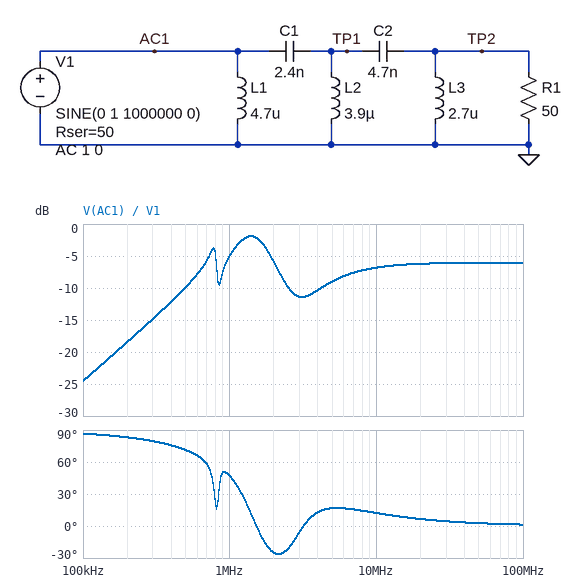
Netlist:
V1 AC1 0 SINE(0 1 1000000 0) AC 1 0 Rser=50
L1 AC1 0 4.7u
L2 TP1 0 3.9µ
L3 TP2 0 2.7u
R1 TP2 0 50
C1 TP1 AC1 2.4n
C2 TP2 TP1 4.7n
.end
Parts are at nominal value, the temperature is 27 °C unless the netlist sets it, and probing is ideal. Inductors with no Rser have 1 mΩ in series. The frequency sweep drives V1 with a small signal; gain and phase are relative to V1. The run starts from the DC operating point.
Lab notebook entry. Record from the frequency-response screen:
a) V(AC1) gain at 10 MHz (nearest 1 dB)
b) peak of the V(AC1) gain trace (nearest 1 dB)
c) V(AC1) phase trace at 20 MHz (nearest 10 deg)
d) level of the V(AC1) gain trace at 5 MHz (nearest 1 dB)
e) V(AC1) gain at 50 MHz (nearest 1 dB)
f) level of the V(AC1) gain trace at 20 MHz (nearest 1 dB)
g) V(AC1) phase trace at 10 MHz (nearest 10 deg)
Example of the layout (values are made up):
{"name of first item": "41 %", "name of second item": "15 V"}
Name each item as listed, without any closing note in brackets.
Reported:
{"V(AC1) gain at 10 MHz": "-7 dB", "peak of the V(AC1) gain trace": "-2 dB", "V(AC1) phase trace at 20 MHz": "10 deg", "level of the V(AC1) gain trace at 5 MHz": "-9 dB", "V(AC1) gain at 50 MHz": "-6 dB", "level of the V(AC1) gain trace at 20 MHz": "-6 dB", "V(AC1) phase trace at 10 MHz": "10 deg"}
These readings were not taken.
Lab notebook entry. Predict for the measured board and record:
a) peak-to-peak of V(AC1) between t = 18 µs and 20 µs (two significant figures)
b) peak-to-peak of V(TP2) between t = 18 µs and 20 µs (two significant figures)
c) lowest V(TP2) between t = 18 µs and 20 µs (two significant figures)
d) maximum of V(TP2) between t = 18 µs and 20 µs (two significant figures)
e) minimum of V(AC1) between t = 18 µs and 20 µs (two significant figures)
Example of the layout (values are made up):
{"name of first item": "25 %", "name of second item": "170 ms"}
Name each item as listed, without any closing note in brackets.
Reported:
{"peak-to-peak of V(AC1) between t = 18 µs and 20 µs": "1.1 V", "peak-to-peak of V(TP2) between t = 18 µs and 20 µs": "510 mV", "lowest V(TP2) between t = 18 µs and 20 µs": "-260 mV", "maximum of V(TP2) between t = 18 µs and 20 µs": "260 mV", "minimum of V(AC1) between t = 18 µs and 20 µs": "-570 mV"}
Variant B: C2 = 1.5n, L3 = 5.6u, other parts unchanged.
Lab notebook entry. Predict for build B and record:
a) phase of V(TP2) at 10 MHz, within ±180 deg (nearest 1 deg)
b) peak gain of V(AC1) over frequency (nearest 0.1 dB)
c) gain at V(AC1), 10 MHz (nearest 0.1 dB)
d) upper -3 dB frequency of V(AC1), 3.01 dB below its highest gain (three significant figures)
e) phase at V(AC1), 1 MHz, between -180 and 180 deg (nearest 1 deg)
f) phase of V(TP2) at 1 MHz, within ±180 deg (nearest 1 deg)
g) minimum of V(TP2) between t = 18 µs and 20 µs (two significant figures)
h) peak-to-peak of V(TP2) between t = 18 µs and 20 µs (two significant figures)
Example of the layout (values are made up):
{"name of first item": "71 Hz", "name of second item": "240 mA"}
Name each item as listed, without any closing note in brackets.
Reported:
{"phase of V(TP2) at 10 MHz, within ±180 deg": "25 deg", "peak gain of V(AC1) over frequency": "-1.1 dB", "gain at V(AC1), 10 MHz": "-6.2 dB", "upper -3 dB frequency of V(AC1), 3.01 dB below its highest gain": "1.08 MHz", "phase at V(AC1), 1 MHz, between -180 and 180 deg": "8 deg", "phase of V(TP2) at 1 MHz, within ±180 deg": "-48 deg", "minimum of V(TP2) between t = 18 µs and 20 µs": "-320 mV", "peak-to-peak of V(TP2) between t = 18 µs and 20 µs": "630 mV"}
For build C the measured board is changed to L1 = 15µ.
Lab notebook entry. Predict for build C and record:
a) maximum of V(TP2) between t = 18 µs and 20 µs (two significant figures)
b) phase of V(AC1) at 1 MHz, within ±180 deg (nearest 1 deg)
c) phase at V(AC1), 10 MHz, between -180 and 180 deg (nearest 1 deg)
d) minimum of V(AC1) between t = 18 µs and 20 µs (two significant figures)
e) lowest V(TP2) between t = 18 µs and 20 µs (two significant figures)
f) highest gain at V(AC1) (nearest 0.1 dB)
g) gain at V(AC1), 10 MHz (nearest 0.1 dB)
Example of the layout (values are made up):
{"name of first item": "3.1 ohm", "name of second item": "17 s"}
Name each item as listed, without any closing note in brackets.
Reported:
{"maximum of V(TP2) between t = 18 µs and 20 µs": "370 mV", "phase of V(AC1) at 1 MHz, within ±180 deg": "6 deg", "phase at V(AC1), 10 MHz, between -180 and 180 deg": "9 deg", "minimum of V(AC1) between t = 18 µs and 20 µs": "-830 mV", "lowest V(TP2) between t = 18 µs and 20 µs": "-370 mV", "highest gain at V(AC1)": "-0.1 dB", "gain at V(AC1), 10 MHz": "-6.7 dB"}
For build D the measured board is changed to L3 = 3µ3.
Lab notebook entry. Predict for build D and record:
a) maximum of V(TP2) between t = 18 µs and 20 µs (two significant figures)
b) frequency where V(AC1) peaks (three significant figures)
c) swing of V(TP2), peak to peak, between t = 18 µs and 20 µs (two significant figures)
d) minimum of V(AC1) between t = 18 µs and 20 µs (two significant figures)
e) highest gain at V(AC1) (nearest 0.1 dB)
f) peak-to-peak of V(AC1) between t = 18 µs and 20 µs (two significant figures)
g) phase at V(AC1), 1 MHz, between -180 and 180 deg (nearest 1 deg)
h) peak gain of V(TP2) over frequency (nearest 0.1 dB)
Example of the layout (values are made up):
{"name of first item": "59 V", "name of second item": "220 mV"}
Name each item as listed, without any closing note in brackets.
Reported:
{"maximum of V(TP2) between t = 18 µs and 20 µs": "280 mV", "frequency where V(AC1) peaks": "1.35 MHz", "swing of V(TP2), peak to peak, between t = 18 µs and 20 µs": "550 mV", "minimum of V(AC1) between t = 18 µs and 20 µs": "-590 mV", "highest gain at V(AC1)": "-2.2 dB", "peak-to-peak of V(AC1) between t = 18 µs and 20 µs": "1.2 V", "phase at V(AC1), 1 MHz, between -180 and 180 deg": "44 deg", "peak gain of V(TP2) over frequency": "-6.0 dB"}
